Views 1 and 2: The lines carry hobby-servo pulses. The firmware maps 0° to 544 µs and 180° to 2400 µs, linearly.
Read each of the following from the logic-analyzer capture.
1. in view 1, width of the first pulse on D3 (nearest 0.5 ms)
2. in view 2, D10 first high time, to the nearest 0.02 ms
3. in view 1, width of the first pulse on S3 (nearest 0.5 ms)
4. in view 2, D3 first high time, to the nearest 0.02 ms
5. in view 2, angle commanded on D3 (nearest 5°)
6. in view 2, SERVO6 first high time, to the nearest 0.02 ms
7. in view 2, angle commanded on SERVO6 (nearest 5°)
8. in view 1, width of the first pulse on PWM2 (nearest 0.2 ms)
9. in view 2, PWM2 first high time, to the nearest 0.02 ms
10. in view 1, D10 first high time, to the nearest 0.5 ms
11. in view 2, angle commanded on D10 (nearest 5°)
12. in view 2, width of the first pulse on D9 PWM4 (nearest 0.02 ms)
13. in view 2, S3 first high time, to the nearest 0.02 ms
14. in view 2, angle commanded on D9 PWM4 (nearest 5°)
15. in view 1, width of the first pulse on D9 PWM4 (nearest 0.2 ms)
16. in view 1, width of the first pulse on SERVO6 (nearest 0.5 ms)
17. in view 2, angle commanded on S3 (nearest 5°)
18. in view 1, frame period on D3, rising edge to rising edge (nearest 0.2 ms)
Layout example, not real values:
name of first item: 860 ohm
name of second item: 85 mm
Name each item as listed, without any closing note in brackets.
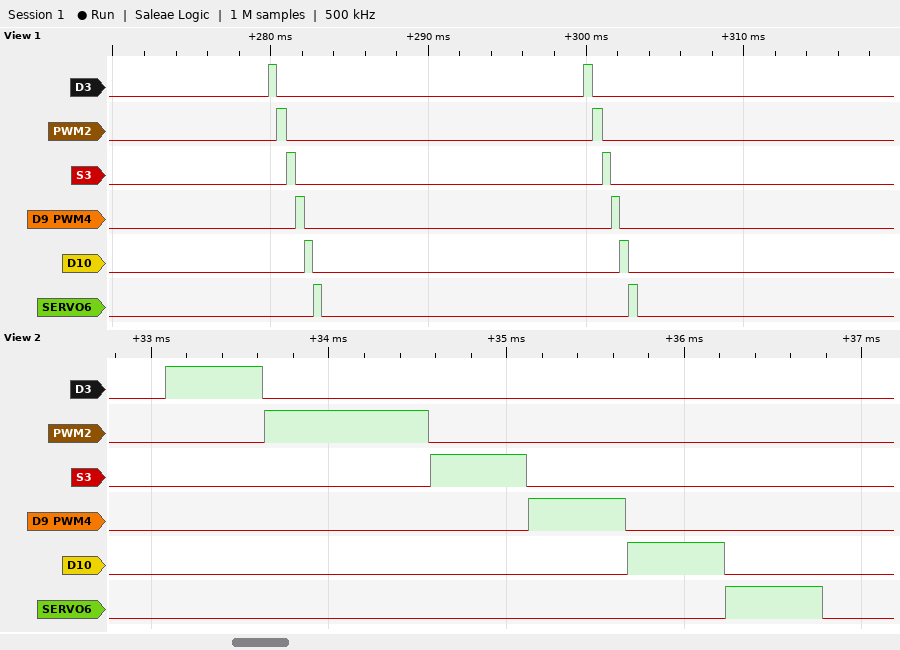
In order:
in view 1, width of the first pulse on D3: 0.5 ms
in view 2, D10 first high time, to the nearest 0.02 ms: 0.54 ms
in view 1, width of the first pulse on S3: 0.5 ms
in view 2, D3 first high time, to the nearest 0.02 ms: 0.54 ms
in view 2, angle commanded on D3: 0°
in view 2, SERVO6 first high time, to the nearest 0.02 ms: 0.54 ms
in view 2, angle commanded on SERVO6: 0°
in view 1, width of the first pulse on PWM2: 0.6 ms
in view 2, PWM2 first high time, to the nearest 0.02 ms: 0.92 ms
in view 1, D10 first high time, to the nearest 0.5 ms: 0.5 ms
in view 2, angle commanded on D10: 0°
in view 2, width of the first pulse on D9 PWM4: 0.54 ms
in view 2, S3 first high time, to the nearest 0.02 ms: 0.54 ms
in view 2, angle commanded on D9 PWM4: 0°
in view 1, width of the first pulse on D9 PWM4: 0.6 ms
in view 1, width of the first pulse on SERVO6: 0.5 ms
in view 2, angle commanded on S3: 0°
in view 1, frame period on D3, rising edge to rising edge: 20.0 ms
